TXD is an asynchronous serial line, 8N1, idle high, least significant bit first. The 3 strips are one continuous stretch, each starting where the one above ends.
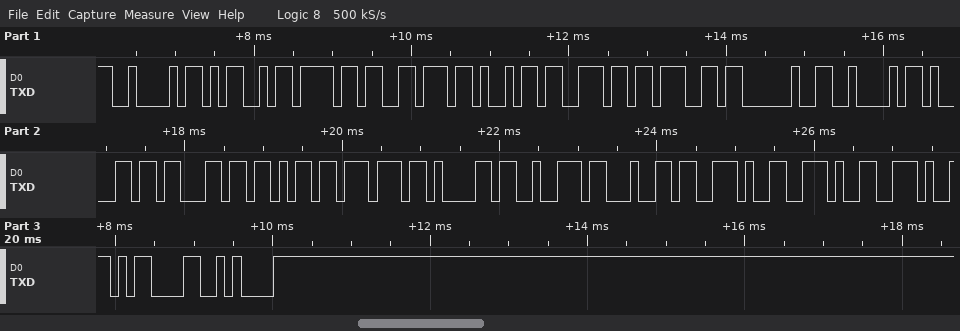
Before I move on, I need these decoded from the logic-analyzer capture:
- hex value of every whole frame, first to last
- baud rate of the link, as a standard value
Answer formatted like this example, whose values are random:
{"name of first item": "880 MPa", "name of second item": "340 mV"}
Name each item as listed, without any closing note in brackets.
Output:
{"hex value of every whole frame, first to last": "0x42 0x4D 0x6F 0x76 0x69 0x6E 0x67 0x20 0x42 0x61 0x63 0x6B 0x77 0x61 0x72 0x64 0x2E 0x2E 0x2E 0x0D 0x0A", "baud rate of the link, as a standard value": "9600 baud"}
